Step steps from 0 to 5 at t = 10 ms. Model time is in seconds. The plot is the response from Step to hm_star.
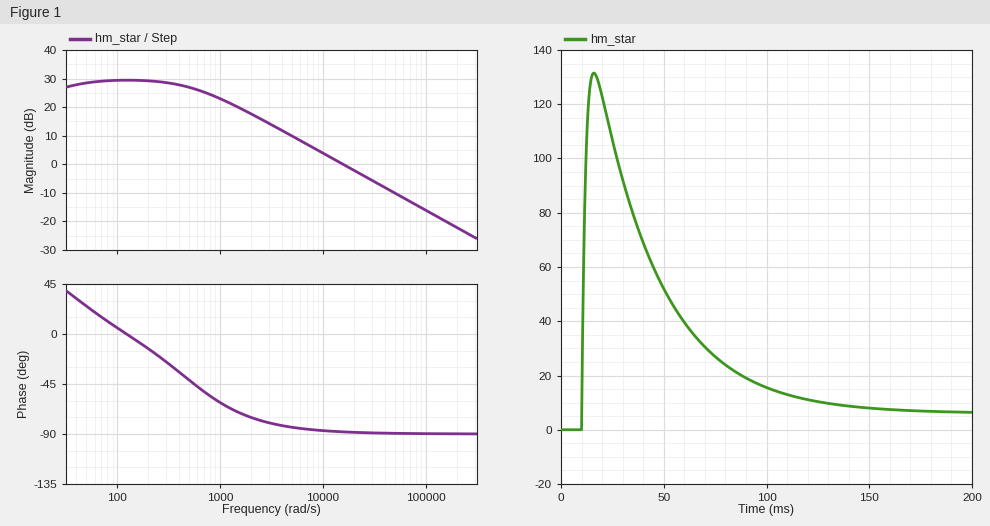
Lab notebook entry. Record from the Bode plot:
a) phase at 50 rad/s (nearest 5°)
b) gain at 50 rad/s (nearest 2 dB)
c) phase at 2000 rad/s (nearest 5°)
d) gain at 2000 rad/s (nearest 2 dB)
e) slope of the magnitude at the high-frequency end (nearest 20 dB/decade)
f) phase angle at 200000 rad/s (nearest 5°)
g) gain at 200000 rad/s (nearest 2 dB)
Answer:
25°
28 dB
-75°
18 dB
-20 dB/decade
-90°
-22 dB
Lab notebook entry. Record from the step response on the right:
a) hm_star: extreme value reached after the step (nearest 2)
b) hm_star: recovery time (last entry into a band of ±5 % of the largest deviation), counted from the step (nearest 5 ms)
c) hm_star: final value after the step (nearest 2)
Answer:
132
100 ms
6
